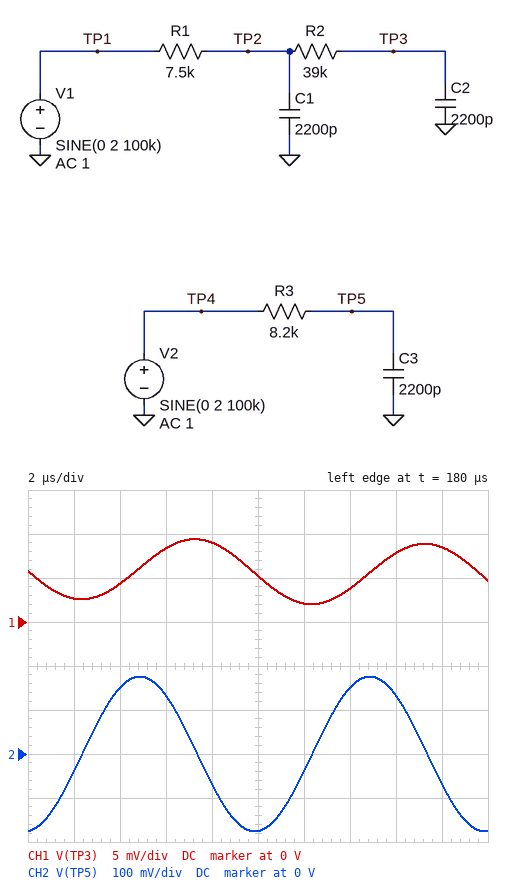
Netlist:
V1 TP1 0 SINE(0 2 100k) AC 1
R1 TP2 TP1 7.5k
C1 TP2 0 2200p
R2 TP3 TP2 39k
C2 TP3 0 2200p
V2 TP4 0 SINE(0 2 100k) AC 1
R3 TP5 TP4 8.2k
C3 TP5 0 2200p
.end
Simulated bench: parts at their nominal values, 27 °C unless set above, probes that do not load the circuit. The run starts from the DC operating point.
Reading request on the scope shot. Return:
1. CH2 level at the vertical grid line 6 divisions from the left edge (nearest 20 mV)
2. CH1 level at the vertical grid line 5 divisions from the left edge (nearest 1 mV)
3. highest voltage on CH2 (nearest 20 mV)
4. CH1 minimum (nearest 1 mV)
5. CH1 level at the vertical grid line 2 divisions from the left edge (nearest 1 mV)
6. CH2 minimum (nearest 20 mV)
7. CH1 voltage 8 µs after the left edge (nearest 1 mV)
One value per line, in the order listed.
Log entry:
-40 mV
5 mV
180 mV
2 mV
4 mV
-180 mV
9 mV
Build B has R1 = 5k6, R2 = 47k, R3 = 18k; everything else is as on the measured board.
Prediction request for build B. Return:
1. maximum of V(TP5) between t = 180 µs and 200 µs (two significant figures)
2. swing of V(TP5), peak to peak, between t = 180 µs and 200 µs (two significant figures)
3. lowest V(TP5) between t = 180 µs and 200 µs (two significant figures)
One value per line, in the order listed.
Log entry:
81 mV
160 mV
-80 mV
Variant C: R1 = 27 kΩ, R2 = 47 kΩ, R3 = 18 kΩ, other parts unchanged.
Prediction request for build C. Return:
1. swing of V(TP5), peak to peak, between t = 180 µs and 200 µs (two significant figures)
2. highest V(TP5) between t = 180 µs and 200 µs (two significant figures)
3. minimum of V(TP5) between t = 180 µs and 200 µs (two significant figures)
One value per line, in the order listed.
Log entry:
160 mV
81 mV
-80 mV
